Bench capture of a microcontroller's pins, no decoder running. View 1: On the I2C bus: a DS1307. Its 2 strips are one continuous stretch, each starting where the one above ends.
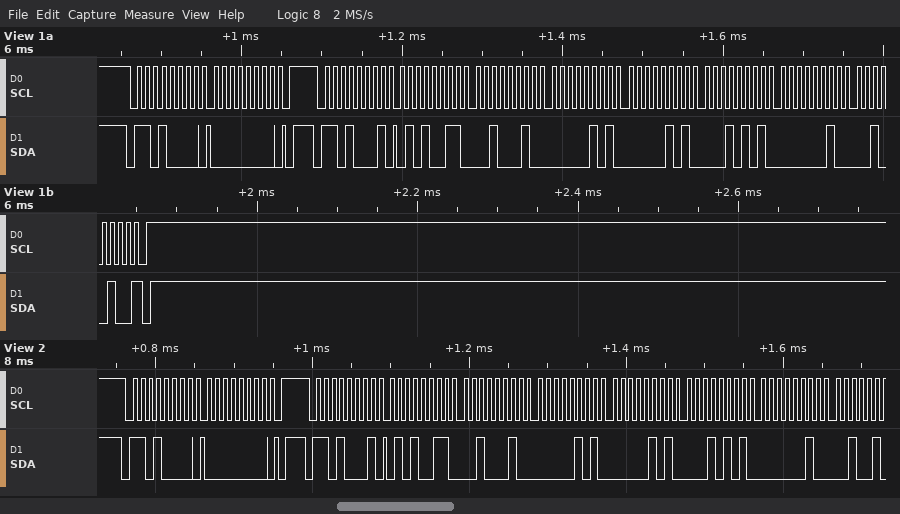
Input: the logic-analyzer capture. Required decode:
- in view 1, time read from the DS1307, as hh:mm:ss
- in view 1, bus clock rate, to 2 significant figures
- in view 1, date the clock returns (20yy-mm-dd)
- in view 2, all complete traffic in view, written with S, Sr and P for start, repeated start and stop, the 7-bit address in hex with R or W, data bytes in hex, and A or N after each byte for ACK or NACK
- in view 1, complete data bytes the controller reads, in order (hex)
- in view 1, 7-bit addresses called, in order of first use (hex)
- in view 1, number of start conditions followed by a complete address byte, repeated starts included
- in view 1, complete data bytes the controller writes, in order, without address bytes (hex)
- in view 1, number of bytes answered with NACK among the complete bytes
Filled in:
05:22:53
100 kHz
2024-02-15
S 68W A 00 A P S 68R A 53 A 22 A 05 A 05 A 15 A 02 A
53 22 05 05 15 02 24
0x68
2
00
1
